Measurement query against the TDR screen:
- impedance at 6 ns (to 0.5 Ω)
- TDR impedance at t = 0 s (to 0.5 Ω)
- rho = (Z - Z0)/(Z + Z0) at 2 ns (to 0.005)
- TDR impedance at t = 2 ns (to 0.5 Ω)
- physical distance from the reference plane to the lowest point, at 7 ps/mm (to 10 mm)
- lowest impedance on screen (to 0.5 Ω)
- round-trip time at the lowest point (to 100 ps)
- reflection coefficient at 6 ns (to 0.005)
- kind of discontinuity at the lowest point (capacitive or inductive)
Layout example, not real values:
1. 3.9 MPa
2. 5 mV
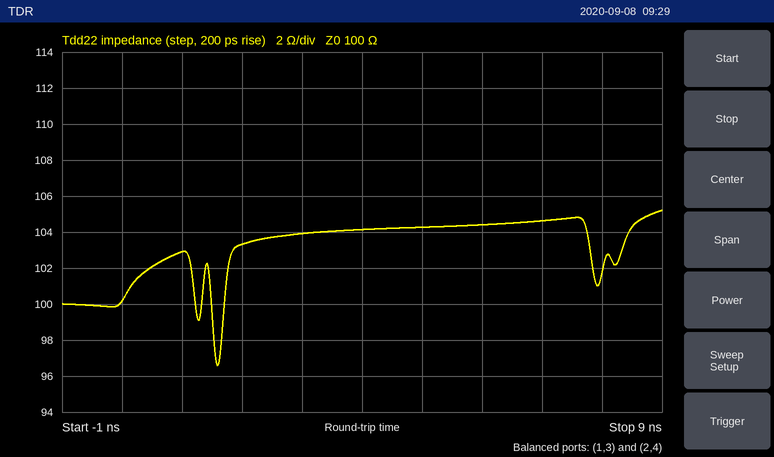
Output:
1. 104.5 Ω
2. 100.0 Ω
3. +0.015
4. 103.5 Ω
5. 110 mm
6. 96.5 Ω
7. 1.6 ns
8. +0.020
9. capacitive
